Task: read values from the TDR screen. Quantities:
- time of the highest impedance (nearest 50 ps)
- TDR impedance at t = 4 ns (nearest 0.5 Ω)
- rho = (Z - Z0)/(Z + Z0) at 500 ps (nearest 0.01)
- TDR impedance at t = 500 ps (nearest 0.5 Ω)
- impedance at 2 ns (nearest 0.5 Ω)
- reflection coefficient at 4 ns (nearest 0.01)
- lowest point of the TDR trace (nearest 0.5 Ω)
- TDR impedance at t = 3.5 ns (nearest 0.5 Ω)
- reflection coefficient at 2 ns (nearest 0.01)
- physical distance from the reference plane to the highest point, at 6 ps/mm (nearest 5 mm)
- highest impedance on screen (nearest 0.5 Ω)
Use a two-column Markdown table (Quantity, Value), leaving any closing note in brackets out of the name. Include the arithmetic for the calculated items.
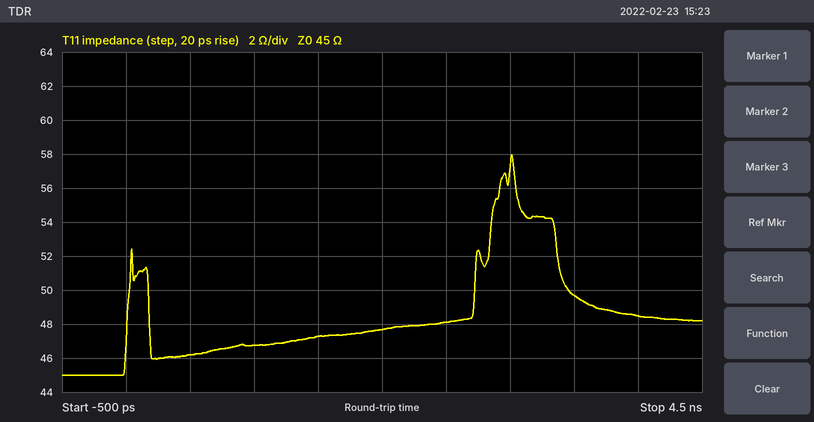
| Quantity | Value |
|---|---|
| time of the highest impedance | 3.00 ns |
| TDR impedance at t = 4 ns | 48.5 Ω |
| rho = (Z - Z0)/(Z + Z0) at 500 ps | (46 − 45)/(46 + 45) ≈ +0.01 |
| TDR impedance at t = 500 ps | 46.0 Ω |
| impedance at 2 ns | 47.5 Ω |
| reflection coefficient at 4 ns | (48.5 − 45)/(48.5 + 45) ≈ +0.04 |
| lowest point of the TDR trace | 45.0 Ω |
| TDR impedance at t = 3.5 ns | 49.5 Ω |
| reflection coefficient at 2 ns | (47.5 − 45)/(47.5 + 45) ≈ +0.03 |
| physical distance from the reference plane to the highest point, at 6 ps/mm | 3.00 ns / 2 / 6 ps/mm ≈ 250 mm |
| highest impedance on screen | 58.0 Ω |
